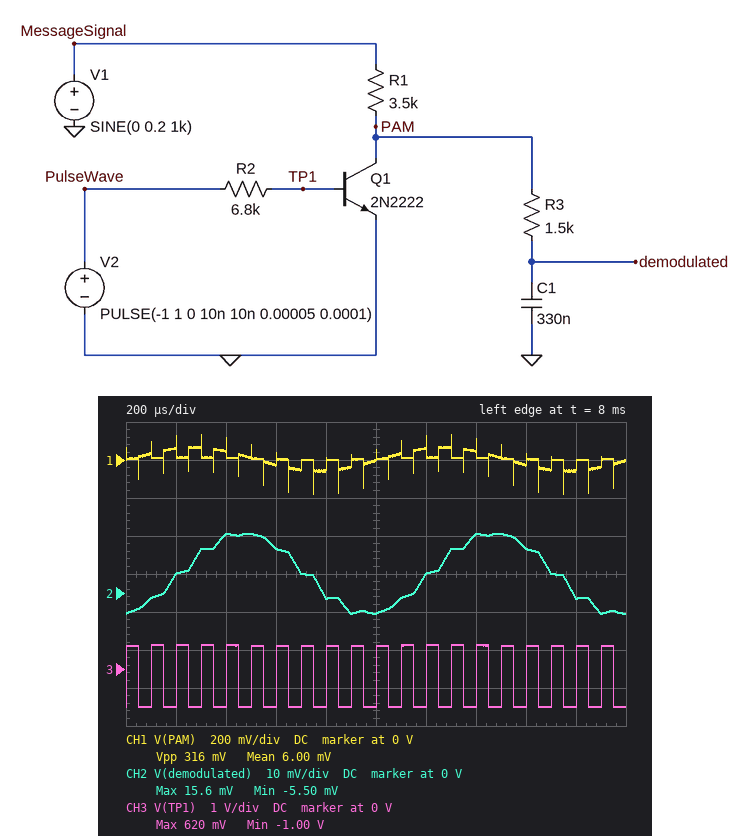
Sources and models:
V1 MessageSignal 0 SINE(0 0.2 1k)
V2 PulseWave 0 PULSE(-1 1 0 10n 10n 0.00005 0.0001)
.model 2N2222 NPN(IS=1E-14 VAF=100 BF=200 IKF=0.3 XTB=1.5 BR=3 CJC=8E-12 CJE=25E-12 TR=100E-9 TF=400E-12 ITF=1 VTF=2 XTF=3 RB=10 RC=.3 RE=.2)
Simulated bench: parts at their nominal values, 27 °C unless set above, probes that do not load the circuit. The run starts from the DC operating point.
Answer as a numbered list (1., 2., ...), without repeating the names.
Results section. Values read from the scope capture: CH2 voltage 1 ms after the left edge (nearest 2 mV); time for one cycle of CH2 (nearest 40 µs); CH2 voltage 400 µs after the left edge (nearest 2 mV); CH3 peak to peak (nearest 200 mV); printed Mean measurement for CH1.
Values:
1. -6 mV
2. 1.00 ms
3. 16 mV
4. 1.6 V
5. 6.00 mV
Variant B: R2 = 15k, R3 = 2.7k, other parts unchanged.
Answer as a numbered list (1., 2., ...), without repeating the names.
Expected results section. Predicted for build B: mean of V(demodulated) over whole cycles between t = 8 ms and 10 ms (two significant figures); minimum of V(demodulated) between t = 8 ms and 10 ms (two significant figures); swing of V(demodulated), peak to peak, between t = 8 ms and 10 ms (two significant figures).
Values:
1. 3.8 mV
2. -5.2 mV
3. 18 mV
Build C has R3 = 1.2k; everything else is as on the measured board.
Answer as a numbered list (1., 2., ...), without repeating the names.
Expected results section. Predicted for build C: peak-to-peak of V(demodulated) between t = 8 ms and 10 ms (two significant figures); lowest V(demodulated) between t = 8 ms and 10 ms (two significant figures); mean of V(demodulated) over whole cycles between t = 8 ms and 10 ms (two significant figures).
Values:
1. 23 mV
2. -6.2 mV
3. 5.3 mV
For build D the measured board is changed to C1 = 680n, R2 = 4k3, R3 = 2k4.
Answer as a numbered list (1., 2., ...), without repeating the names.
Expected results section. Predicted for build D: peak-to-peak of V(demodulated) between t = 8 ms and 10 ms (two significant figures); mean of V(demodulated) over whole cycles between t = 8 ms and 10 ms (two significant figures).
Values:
1. 8.4 mV
2. 4.9 mV
